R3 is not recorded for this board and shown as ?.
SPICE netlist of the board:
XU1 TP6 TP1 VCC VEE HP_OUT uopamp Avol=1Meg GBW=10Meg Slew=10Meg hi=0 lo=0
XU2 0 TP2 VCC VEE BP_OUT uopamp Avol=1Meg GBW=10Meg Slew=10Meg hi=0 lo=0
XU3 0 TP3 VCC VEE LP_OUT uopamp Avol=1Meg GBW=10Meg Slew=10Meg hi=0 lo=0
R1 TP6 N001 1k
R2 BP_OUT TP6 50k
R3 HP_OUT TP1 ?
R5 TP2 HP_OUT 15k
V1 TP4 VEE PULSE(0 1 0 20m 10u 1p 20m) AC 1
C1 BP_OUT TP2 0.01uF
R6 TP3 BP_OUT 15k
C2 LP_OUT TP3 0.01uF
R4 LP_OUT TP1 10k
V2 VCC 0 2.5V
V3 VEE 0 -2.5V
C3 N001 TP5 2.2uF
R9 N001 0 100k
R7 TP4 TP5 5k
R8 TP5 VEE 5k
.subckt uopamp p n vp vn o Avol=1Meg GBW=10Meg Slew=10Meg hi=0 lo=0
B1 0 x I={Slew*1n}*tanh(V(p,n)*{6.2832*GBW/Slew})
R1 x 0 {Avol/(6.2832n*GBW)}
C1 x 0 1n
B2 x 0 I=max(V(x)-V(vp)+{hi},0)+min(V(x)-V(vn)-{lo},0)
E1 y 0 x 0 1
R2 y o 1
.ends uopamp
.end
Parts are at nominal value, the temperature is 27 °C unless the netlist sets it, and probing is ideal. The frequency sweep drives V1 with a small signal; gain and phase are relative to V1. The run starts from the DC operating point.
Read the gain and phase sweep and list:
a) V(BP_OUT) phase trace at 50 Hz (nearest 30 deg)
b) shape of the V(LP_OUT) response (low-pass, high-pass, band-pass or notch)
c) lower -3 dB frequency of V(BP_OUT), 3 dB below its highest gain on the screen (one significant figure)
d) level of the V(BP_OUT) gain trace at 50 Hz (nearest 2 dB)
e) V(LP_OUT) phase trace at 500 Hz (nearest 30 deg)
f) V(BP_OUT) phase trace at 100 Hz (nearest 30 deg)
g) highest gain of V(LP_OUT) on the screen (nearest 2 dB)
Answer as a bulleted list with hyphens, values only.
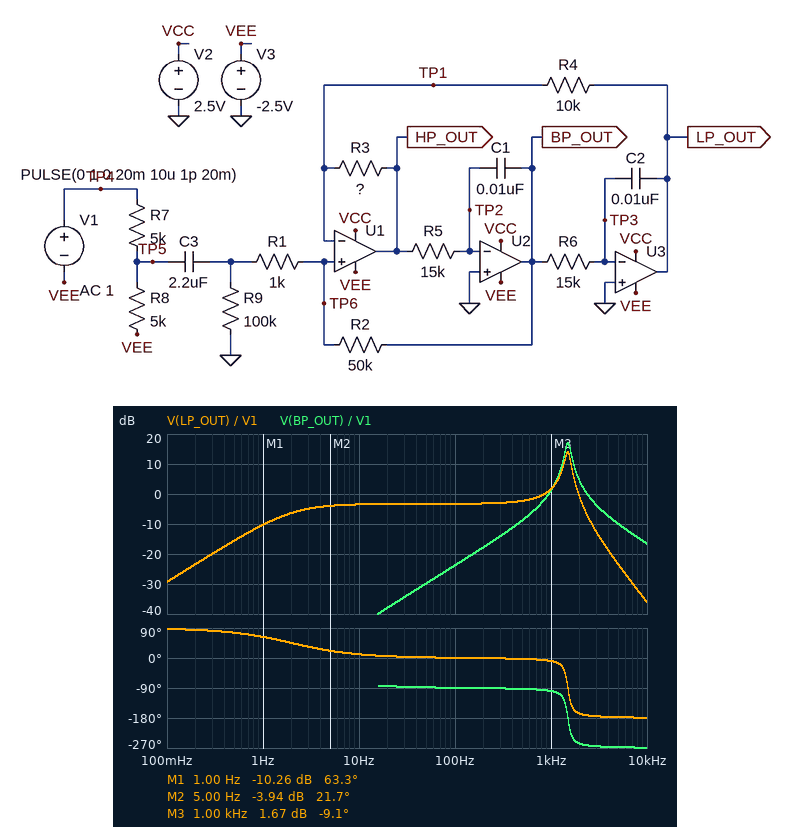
- -90 deg
- band-pass
- 1 kHz
- -30 dB
- 0 deg
- -90 deg
- 14 dB
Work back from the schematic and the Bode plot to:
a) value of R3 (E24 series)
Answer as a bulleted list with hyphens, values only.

- 20 kΩ
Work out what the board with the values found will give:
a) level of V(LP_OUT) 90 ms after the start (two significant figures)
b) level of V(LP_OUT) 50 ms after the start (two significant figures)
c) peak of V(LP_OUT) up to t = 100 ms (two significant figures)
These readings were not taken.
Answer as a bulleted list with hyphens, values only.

- 120 mV
- 200 mV
- 600 mV
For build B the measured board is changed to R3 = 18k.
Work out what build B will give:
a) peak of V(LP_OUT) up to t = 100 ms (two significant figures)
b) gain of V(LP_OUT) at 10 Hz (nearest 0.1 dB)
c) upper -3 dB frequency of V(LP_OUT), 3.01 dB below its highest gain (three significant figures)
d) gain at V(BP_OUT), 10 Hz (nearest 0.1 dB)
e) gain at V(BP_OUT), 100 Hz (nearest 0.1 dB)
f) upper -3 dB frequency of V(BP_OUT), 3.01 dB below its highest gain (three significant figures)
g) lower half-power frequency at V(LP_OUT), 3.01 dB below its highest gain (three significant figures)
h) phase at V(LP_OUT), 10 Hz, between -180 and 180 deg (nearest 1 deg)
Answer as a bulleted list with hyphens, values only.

- 630 mV
- -3.2 dB
- 1.51 kHz
- -43.7 dB
- -23.5 dB
- 1.52 kHz
- 1.32 kHz
- 11 deg
